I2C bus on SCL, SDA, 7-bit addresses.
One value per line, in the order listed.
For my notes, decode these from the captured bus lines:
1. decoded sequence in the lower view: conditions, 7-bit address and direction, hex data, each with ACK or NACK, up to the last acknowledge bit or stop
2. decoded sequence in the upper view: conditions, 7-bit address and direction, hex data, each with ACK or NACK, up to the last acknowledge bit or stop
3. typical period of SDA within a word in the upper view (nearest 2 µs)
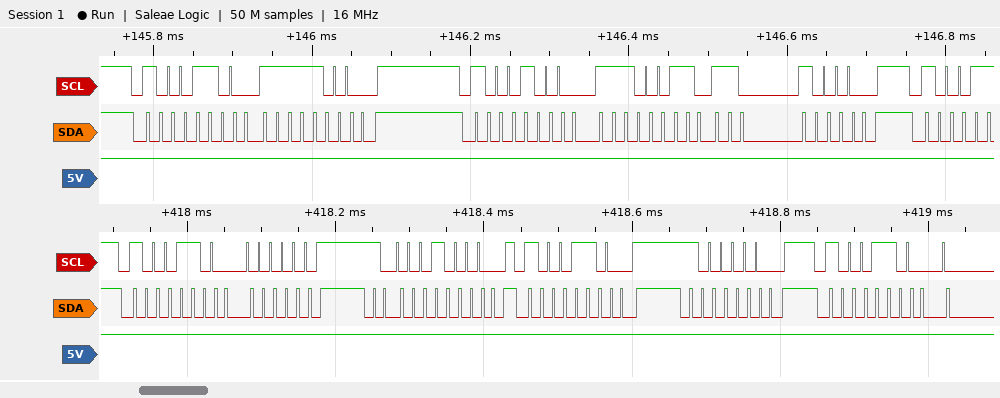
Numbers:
start, address 46 write ACK, 03 ACK, 10 ACK, stop, start, address 46 write ACK, C0 ACK, stop, start, address 46 write ACK
start, address 46 write ACK, F8 ACK, stop, start, address 44 write ACK, E3 ACK, D0 ACK, stop
16 µs
